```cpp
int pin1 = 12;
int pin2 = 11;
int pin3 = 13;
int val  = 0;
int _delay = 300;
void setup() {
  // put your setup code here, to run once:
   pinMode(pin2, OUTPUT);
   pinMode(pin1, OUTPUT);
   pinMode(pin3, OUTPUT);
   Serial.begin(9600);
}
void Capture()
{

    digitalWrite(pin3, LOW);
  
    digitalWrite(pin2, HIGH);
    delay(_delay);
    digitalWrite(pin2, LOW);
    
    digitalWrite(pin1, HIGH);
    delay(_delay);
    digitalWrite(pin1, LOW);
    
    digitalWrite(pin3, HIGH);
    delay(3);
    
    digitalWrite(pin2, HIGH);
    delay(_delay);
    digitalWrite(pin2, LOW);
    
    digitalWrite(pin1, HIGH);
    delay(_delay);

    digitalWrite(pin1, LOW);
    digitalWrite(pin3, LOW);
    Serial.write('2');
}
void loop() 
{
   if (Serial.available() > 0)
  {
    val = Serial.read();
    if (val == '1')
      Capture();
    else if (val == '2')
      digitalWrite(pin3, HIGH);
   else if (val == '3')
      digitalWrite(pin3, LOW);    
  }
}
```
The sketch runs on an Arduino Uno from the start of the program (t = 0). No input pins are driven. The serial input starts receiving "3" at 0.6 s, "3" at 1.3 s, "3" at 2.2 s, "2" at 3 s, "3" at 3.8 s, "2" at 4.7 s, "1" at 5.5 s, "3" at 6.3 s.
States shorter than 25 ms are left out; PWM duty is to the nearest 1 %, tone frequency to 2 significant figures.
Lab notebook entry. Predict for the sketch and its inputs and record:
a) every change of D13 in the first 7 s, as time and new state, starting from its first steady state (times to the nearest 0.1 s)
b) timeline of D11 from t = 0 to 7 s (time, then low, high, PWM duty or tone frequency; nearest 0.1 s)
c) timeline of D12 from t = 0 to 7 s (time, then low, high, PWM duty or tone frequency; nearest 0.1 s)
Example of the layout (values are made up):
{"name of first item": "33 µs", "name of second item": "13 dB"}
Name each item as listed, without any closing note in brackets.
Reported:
{"every change of D13 in the first 7 s, as time and new state, starting from its first steady state": "0 s low; 3 s high; 3.8 s low; 4.7 s high; 5.5 s low; 6.1 s high; 6.7 s low", "timeline of D11 from t = 0 to 7 s": "0 s low; 5.5 s high; 5.8 s low; 6.1 s high; 6.4 s low", "timeline of D12 from t = 0 to 7 s": "0 s low; 5.8 s high; 6.1 s low; 6.4 s high; 6.7 s low"}
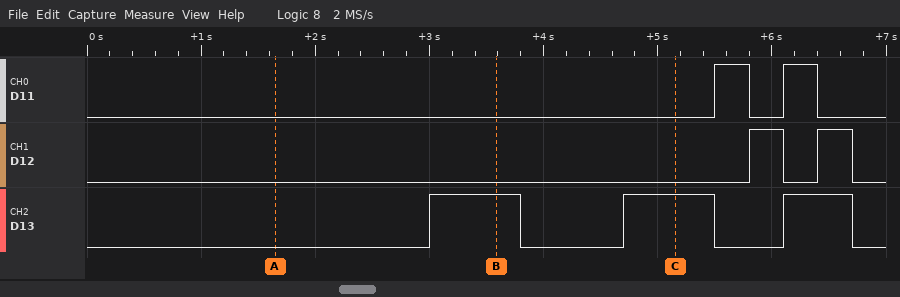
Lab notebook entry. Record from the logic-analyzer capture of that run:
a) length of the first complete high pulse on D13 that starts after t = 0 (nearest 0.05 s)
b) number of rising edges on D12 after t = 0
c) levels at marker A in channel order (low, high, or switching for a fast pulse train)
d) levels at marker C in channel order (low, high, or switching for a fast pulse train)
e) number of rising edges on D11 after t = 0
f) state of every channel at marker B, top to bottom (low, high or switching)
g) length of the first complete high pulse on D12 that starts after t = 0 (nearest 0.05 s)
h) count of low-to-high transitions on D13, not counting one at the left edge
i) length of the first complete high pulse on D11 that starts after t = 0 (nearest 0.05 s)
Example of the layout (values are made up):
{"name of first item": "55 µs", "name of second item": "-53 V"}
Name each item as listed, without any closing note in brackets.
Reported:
{"length of the first complete high pulse on D13 that starts after t = 0": "0.80 s", "number of rising edges on D12 after t = 0": "2", "levels at marker A in channel order": "D11 low, D12 low, D13 low", "levels at marker C in channel order": "D11 low, D12 low, D13 high", "number of rising edges on D11 after t = 0": "2", "state of every channel at marker B, top to bottom": "D11 low, D12 low, D13 high", "length of the first complete high pulse on D12 that starts after t = 0": "0.30 s", "count of low-to-high transitions on D13, not counting one at the left edge": "3", "length of the first complete high pulse on D11 that starts after t = 0": "0.30 s"}
